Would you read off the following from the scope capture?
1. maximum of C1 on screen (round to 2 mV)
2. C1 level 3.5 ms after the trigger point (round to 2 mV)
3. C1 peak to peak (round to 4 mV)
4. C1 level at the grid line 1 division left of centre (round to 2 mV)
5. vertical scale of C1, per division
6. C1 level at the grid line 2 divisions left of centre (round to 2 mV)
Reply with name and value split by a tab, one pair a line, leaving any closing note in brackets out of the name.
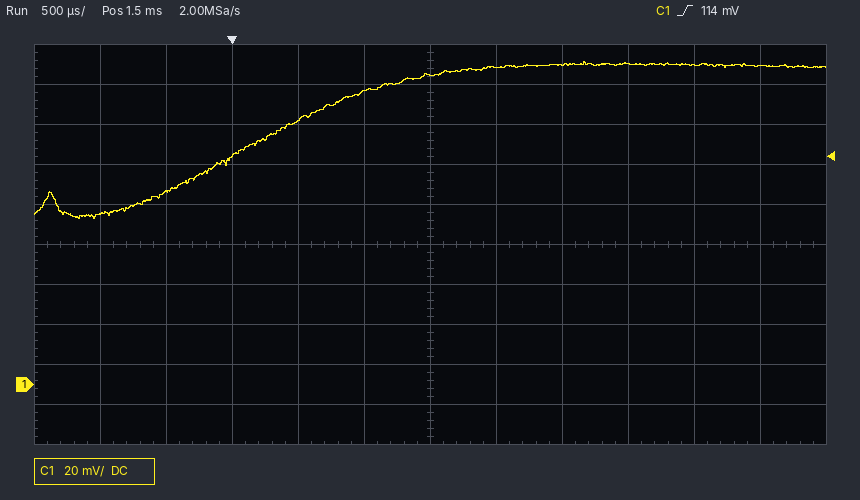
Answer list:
maximum of C1 on screen	162 mV
C1 level 3.5 ms after the trigger point	160 mV
C1 peak to peak	80 mV
C1 level at the grid line 1 division left of centre	146 mV
vertical scale of C1, per division	20 mV
C1 level at the grid line 2 divisions left of centre	132 mV
